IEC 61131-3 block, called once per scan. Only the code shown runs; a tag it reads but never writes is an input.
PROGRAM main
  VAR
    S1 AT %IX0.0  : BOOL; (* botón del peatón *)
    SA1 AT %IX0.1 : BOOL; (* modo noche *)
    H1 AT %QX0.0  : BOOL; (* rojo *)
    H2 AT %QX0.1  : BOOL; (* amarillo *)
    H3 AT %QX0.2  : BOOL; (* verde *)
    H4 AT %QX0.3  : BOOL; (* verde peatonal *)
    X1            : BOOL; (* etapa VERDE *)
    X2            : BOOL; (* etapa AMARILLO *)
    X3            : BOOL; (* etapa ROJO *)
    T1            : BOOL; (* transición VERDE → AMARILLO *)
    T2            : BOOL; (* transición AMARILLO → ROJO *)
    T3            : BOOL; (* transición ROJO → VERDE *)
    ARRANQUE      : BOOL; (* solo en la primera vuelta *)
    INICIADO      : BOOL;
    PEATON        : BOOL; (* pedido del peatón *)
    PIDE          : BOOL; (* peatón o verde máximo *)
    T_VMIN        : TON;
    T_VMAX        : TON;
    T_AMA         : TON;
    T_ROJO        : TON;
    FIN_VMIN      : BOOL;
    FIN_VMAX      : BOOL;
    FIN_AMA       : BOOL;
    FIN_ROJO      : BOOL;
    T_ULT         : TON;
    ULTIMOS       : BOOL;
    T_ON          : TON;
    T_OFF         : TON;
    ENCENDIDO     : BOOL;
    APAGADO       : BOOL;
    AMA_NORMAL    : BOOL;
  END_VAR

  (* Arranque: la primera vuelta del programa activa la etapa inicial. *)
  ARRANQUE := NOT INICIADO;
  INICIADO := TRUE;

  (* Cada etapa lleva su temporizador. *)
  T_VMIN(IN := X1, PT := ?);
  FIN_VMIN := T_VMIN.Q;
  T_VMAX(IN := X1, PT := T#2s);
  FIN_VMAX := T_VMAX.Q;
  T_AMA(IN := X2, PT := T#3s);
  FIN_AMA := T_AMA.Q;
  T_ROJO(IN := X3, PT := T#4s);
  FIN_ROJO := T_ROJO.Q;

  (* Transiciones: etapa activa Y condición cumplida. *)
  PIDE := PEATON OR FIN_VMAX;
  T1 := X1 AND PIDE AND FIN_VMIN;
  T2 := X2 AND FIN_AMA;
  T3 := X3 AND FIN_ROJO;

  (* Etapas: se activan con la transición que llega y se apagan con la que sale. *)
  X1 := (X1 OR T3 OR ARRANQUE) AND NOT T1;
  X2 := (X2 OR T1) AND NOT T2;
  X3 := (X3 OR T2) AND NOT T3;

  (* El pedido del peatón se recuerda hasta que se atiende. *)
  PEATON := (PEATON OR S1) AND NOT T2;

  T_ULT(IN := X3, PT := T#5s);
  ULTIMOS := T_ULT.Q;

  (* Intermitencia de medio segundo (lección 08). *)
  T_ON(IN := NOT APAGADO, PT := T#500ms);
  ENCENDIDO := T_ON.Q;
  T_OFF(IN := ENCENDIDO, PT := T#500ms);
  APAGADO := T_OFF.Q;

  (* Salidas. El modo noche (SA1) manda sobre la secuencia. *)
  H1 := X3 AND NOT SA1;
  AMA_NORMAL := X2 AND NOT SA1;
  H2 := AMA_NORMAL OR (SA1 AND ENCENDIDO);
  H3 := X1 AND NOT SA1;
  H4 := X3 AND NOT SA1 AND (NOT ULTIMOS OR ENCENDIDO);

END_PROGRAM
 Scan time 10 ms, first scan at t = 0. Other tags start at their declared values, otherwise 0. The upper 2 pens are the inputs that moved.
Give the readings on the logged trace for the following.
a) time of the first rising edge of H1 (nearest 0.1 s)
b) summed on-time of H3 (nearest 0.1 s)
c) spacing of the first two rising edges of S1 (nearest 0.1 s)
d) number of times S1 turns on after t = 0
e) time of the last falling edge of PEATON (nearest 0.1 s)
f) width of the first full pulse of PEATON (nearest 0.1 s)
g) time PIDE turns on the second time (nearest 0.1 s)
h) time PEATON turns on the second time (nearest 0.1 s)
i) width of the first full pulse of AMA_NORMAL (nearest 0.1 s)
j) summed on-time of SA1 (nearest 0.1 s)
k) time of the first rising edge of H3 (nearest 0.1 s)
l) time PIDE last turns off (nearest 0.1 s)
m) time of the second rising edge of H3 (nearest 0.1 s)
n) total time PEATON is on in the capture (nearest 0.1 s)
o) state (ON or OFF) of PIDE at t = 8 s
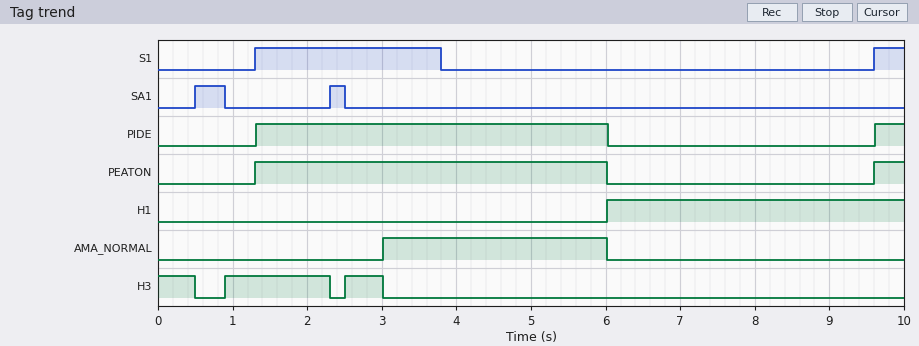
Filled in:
6.0 s
2.4 s
8.3 s
2
6.0 s
4.7 s
9.6 s
9.6 s
3.0 s
0.6 s
0.9 s
6.0 s
2.5 s
5.1 s
OFF
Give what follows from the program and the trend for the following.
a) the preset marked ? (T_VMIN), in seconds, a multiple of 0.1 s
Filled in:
3.0 s
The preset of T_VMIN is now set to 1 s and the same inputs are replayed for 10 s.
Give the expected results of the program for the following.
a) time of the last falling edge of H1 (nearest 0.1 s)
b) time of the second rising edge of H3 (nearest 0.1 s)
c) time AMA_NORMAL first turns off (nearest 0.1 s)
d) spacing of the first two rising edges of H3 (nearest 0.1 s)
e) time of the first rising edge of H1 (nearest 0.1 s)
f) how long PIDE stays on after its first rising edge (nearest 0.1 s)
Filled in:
8.3 s
8.3 s
2.3 s
7.4 s
4.3 s
3.0 s
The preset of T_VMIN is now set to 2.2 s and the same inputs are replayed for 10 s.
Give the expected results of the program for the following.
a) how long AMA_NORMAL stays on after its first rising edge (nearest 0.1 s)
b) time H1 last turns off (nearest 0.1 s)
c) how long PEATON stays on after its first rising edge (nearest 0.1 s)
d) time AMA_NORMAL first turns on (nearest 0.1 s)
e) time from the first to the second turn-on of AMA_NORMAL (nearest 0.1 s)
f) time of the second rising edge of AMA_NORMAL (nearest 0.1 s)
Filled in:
0.1 s
9.2 s
3.9 s
2.2 s
0.3 s
2.5 s
